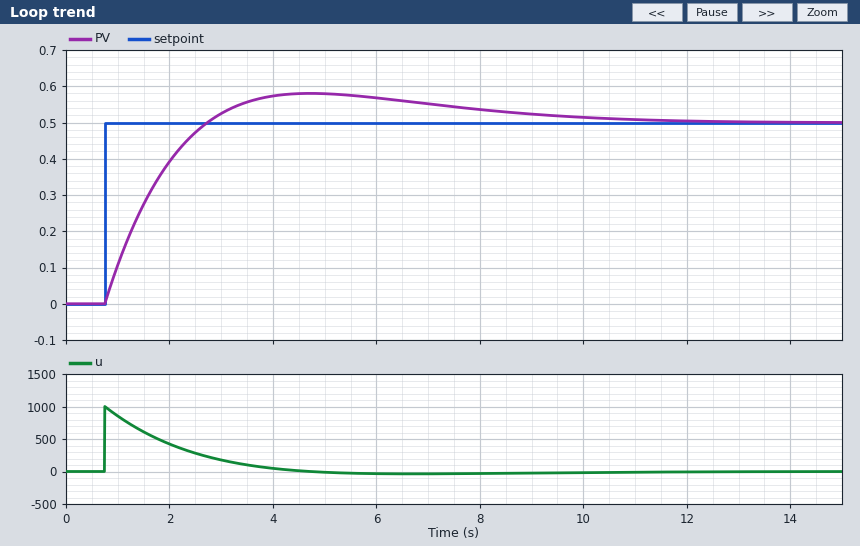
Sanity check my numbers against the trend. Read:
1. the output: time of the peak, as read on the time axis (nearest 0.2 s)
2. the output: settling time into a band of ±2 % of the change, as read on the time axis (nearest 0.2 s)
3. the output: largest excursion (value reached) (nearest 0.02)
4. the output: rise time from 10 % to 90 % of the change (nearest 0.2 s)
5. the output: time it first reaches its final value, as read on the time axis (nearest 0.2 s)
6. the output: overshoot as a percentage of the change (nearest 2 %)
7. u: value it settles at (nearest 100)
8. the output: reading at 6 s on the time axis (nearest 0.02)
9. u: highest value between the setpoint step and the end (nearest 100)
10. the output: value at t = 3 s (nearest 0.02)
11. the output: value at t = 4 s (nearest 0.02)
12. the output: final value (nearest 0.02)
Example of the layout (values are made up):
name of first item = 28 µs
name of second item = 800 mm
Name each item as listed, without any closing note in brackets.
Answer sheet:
the output: time of the peak, as read on the time axis = 4.8 s
the output: settling time into a band of ±2 % of the change, as read on the time axis = 10.6 s
the output: largest excursion (value reached) = 0.58
the output: rise time from 10 % to 90 % of the change = 1.4 s
the output: time it first reaches its final value, as read on the time axis = 2.8 s
the output: overshoot as a percentage of the change = 16 %
u: value it settles at = 0
the output: reading at 6 s on the time axis = 0.56
u: highest value between the setpoint step and the end = 1000
the output: value at t = 3 s = 0.52
the output: value at t = 4 s = 0.58
the output: final value = 0.50
